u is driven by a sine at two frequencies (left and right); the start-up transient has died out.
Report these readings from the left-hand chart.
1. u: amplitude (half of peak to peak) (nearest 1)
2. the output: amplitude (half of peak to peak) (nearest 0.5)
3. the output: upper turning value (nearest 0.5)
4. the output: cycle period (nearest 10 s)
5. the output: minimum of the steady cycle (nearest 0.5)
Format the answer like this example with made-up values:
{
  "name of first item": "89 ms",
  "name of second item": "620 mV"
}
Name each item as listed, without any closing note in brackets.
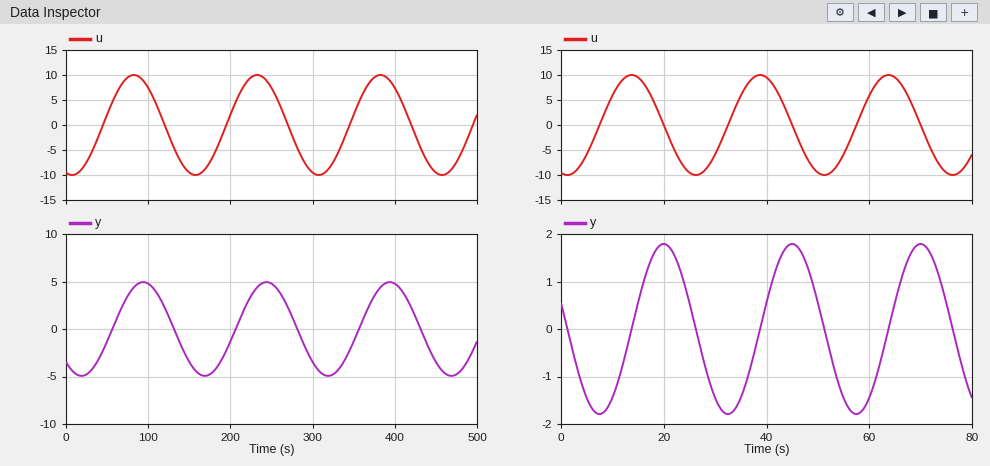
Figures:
{
  "u: amplitude (half of peak to peak)": "10",
  "the output: amplitude (half of peak to peak)": "5.0",
  "the output: upper turning value": "5.0",
  "the output: cycle period": "150 s",
  "the output: minimum of the steady cycle": "-5.0"
}
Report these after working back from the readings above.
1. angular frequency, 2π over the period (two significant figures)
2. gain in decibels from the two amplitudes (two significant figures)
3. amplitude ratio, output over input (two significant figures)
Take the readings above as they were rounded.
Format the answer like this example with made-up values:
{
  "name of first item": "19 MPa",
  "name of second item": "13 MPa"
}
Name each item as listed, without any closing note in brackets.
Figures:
{
  "angular frequency, 2π over the period": "0.042 rad/s",
  "gain in decibels from the two amplitudes": "-6.0 dB",
  "amplitude ratio, output over input": "0.50"
}
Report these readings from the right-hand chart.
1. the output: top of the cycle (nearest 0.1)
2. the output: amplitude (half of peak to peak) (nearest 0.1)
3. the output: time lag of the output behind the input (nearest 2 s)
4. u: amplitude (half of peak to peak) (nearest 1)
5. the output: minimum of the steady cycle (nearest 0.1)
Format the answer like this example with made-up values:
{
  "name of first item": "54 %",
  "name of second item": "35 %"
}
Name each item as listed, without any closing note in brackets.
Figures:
{
  "the output: top of the cycle": "1.8",
  "the output: amplitude (half of peak to peak)": "1.8",
  "the output: time lag of the output behind the input": "6 s",
  "u: amplitude (half of peak to peak)": "10",
  "the output: minimum of the steady cycle": "-1.8"
}
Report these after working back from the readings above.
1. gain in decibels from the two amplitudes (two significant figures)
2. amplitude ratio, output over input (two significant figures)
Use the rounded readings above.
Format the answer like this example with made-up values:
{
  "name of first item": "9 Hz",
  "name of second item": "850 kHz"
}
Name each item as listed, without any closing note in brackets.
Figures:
{
  "gain in decibels from the two amplitudes": "-15 dB",
  "amplitude ratio, output over input": "0.18"
}
